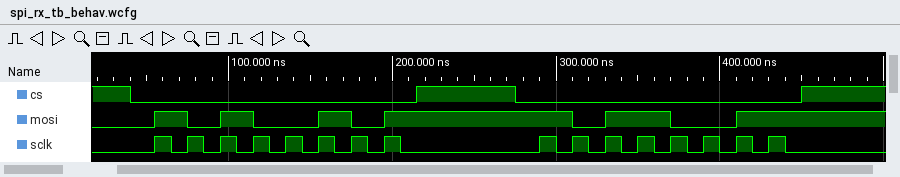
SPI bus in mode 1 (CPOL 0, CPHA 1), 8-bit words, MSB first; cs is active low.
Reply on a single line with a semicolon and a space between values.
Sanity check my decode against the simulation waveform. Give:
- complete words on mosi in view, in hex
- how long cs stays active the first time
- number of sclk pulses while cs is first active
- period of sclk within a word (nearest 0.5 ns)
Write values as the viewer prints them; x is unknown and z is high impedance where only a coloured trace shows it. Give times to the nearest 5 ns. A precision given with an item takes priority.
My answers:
A5, B3; 175 ns; 8; 20 ns
